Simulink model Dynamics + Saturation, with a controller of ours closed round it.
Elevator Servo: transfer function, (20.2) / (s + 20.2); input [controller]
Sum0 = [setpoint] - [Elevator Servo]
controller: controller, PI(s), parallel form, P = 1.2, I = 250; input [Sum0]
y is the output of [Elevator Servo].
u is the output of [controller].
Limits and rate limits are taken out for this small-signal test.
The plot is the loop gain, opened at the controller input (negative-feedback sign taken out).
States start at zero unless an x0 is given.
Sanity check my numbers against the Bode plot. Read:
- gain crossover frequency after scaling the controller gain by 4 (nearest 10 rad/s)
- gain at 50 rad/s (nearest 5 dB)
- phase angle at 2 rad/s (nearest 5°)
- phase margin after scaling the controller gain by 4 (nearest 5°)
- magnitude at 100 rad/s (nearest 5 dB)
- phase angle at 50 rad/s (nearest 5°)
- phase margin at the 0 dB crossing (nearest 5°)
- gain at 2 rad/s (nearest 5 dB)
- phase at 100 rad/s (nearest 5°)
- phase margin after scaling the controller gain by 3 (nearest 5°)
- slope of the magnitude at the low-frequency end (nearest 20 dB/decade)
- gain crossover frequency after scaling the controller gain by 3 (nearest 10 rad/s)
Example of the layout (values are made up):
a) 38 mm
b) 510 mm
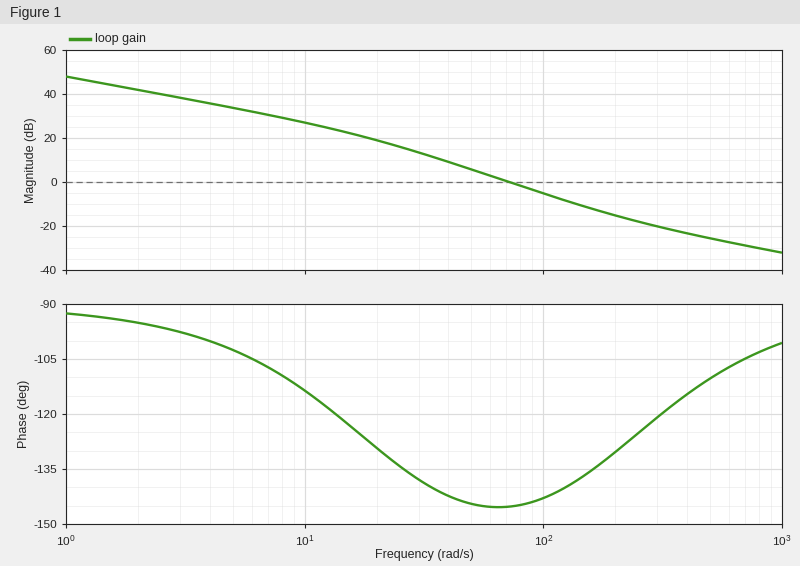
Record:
a) 160 rad/s
b) 5 dB
c) -95°
d) 45°
e) -5 dB
f) -145°
g) 35°
h) 40 dB
i) -145°
j) 40°
k) -20 dB/decade
l) 130 rad/s
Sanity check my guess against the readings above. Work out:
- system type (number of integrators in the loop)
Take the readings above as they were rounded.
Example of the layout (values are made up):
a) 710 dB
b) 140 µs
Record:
a) 1
